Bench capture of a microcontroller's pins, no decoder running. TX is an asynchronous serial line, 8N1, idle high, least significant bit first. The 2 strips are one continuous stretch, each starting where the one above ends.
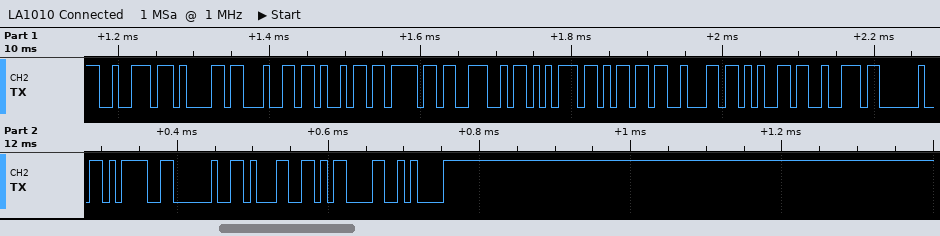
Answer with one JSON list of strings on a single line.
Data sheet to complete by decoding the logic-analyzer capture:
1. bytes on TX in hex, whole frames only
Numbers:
["0x72 0x61 0x64 0x69 0x6F 0x4E 0x75 0x6D 0x62 0x65 0x72 0x20 0x3D 0x20 0x31 0x0D 0x0A"]
